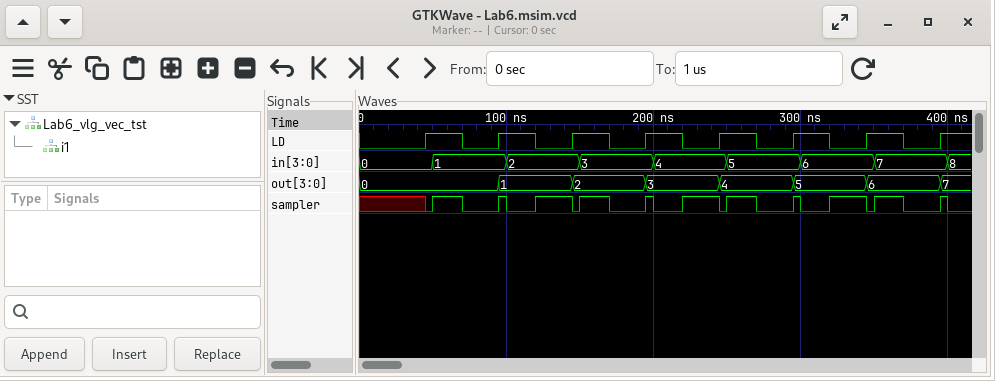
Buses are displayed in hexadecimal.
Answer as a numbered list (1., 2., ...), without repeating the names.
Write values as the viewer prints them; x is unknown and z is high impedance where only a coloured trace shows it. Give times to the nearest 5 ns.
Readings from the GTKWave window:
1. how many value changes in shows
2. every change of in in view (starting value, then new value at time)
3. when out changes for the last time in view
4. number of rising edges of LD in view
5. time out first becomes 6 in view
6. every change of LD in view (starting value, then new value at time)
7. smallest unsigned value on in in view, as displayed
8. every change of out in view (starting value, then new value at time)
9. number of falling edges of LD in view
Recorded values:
1. 8
2. 0, 1 at 50 ns, 2 at 100 ns, 3 at 150 ns, 4 at 200 ns, 5 at 250 ns, 6 at 300 ns, 7 at 350 ns, 8 at 400 ns
3. 395 ns
4. 8
5. 345 ns
6. 0, 1 at 45 ns, 0 at 70 ns, 1 at 95 ns, 0 at 120 ns, 1 at 145 ns, 0 at 170 ns, 1 at 195 ns, 0 at 220 ns, 1 at 245 ns, 0 at 270 ns, 1 at 295 ns, 0 at 320 ns, 1 at 345 ns, 0 at 370 ns, 1 at 395 ns
7. 0
8. 0, 1 at 95 ns, 2 at 145 ns, 3 at 195 ns, 4 at 245 ns, 5 at 295 ns, 6 at 345 ns, 7 at 395 ns
9. 7
